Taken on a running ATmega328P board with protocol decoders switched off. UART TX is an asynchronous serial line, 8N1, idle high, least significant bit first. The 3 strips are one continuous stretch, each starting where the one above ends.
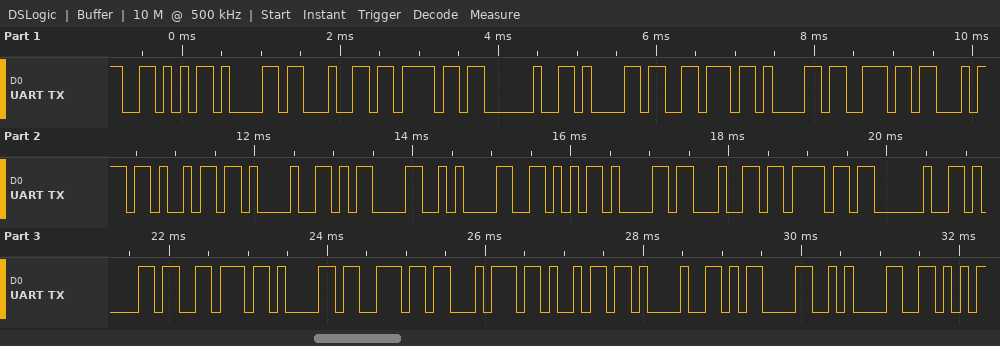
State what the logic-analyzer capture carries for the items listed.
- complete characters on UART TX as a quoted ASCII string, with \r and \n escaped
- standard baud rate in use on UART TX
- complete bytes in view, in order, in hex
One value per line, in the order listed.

"Vado avanti!\r\nVado avanti!\r\nV"
9600 baud
56 61 64 6F 20 61 76 61 6E 74 69 21 0D 0A 56 61 64 6F 20 61 76 61 6E 74 69 21 0D 0A 56
